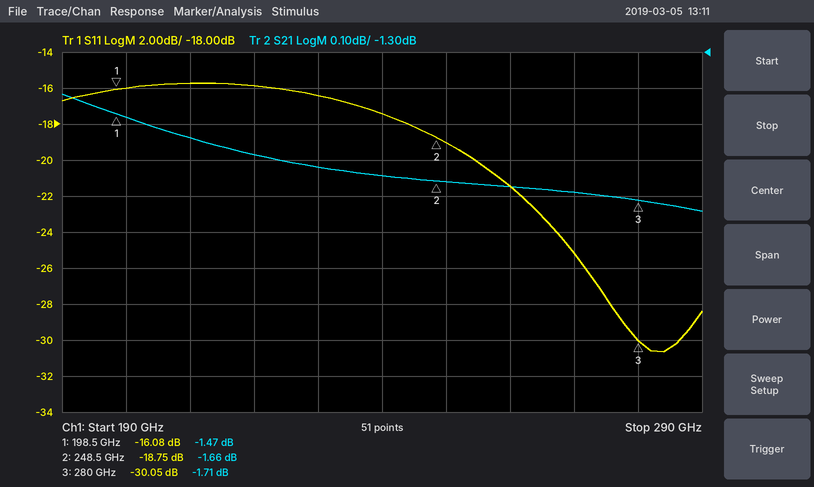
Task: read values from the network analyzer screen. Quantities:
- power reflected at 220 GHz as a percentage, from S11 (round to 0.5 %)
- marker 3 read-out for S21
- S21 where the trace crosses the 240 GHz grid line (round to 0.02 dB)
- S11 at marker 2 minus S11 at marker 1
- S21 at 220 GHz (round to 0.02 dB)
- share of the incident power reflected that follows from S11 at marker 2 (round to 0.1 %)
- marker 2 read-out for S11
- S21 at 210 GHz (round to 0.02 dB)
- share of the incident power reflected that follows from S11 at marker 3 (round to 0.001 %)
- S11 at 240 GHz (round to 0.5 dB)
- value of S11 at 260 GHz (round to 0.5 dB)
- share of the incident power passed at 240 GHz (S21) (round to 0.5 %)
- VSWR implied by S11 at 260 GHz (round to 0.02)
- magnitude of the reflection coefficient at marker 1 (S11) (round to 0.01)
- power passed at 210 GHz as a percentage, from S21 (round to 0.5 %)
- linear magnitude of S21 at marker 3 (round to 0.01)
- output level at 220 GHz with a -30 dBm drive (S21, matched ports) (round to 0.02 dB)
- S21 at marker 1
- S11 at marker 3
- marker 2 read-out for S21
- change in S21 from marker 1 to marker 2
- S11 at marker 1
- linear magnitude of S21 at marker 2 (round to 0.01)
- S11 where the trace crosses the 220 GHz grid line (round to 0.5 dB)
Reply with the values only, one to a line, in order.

2.5 %
-1.71 dB
-1.64 dB
-2.67 dB
-1.58 dB
1.3 %
-18.75 dB
-1.54 dB
0.099 %
-17.5 dB
-21.5 dB
68.5 %
1.18
0.16
70.0 %
0.82
-31.58 dBm
-1.47 dB
-30.05 dB
-1.66 dB
-0.19 dB
-16.08 dB
0.83
-16.0 dB
